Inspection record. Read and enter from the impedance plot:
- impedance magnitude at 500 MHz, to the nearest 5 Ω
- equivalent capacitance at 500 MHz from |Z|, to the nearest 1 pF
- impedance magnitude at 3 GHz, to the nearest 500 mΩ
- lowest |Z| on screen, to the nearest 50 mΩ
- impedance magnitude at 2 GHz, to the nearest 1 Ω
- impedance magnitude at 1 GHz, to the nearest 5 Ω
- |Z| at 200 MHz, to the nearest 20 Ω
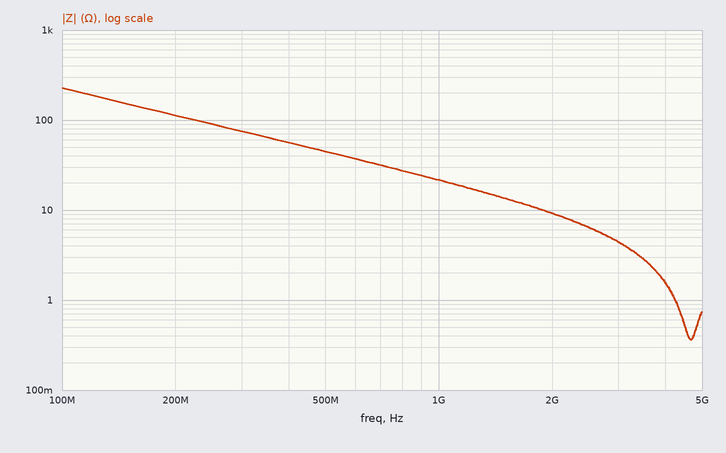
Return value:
45 Ω
7 pF
4.5 Ω
350 mΩ
9 Ω
20 Ω
120 Ω
